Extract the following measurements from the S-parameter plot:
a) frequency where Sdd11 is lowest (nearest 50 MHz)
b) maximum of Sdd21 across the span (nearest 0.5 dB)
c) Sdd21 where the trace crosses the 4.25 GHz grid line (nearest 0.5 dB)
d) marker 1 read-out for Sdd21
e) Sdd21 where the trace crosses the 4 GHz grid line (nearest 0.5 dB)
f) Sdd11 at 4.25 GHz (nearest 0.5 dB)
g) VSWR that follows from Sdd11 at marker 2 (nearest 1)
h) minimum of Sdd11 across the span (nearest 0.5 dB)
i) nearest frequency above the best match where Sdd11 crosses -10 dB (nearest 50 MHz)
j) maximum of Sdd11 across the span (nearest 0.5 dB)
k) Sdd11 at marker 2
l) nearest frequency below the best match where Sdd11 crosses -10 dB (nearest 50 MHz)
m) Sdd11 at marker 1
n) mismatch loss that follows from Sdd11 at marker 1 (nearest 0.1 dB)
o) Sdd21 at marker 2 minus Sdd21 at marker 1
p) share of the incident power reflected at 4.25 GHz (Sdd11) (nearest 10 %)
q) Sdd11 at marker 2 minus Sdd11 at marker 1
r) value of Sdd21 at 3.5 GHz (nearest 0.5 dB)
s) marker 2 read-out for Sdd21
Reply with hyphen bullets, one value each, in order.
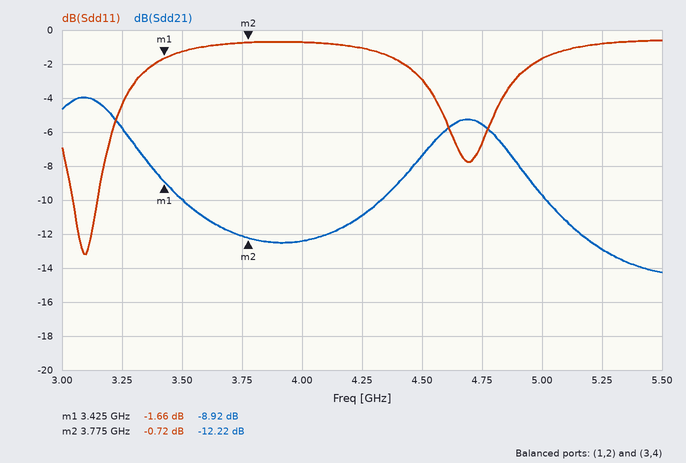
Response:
- 3.10 GHz
- -4.0 dB
- -11.0 dB
- -8.92 dB
- -12.5 dB
- -1.0 dB
- 24
- -13.0 dB
- 3.15 GHz
- -0.5 dB
- -0.72 dB
- 3.05 GHz
- -1.66 dB
- 5.0 dB
- -3.30 dB
- 80 %
- 0.94 dB
- -10.0 dB
- -12.22 dB
